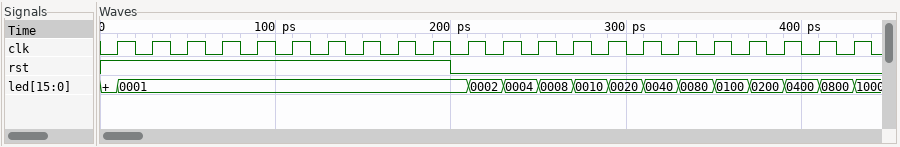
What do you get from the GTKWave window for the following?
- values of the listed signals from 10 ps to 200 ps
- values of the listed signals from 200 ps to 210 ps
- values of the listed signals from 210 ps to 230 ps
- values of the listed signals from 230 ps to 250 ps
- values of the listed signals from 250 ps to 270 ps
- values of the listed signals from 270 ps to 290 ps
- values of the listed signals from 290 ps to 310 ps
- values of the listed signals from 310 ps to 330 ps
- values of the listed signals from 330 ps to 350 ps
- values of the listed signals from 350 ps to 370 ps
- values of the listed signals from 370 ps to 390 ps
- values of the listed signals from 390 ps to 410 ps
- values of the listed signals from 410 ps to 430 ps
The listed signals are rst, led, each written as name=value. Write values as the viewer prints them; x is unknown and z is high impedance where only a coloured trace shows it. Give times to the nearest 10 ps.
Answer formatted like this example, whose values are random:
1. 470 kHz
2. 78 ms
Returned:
1. rst=1, led=0001
2. rst=0, led=0001
3. rst=0, led=0002
4. rst=0, led=0004
5. rst=0, led=0008
6. rst=0, led=0010
7. rst=0, led=0020
8. rst=0, led=0040
9. rst=0, led=0080
10. rst=0, led=0100
11. rst=0, led=0200
12. rst=0, led=0400
13. rst=0, led=0800
